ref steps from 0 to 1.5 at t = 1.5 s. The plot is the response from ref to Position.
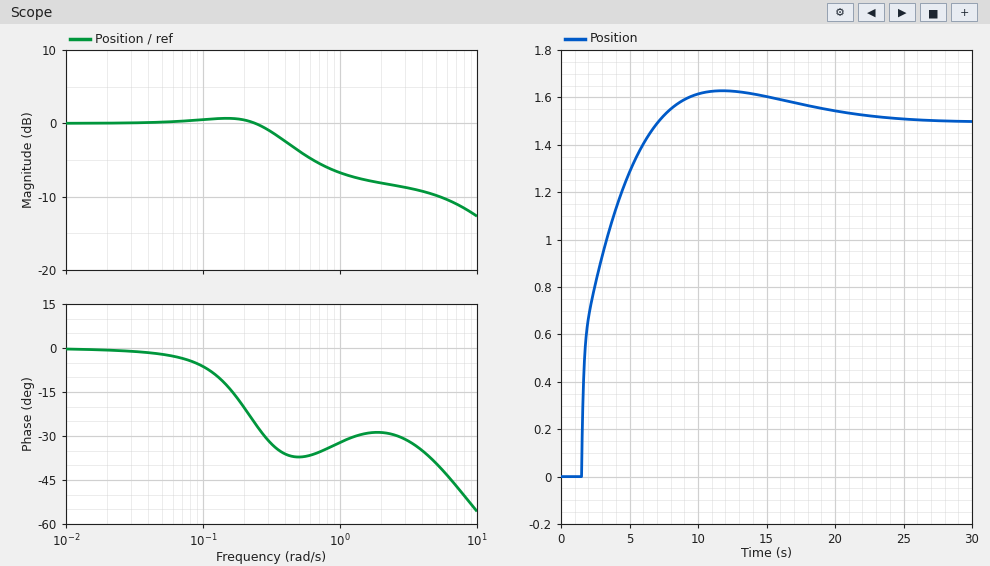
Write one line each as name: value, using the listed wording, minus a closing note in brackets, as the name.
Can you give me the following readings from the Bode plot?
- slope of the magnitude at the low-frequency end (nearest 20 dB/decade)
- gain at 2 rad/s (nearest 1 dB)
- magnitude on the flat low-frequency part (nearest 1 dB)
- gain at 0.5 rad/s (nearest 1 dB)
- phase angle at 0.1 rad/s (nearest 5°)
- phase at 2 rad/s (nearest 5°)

slope of the magnitude at the low-frequency end: 0 dB/decade
gain at 2 rad/s: -8 dB
magnitude on the flat low-frequency part: 0 dB
gain at 0.5 rad/s: -4 dB
phase angle at 0.1 rad/s: -5°
phase at 2 rad/s: -30°
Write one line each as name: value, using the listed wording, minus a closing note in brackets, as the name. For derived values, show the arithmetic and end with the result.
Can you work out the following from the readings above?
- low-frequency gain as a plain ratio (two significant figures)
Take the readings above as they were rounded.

low-frequency gain as a plain ratio: 10^(0 / 20) = 1.0
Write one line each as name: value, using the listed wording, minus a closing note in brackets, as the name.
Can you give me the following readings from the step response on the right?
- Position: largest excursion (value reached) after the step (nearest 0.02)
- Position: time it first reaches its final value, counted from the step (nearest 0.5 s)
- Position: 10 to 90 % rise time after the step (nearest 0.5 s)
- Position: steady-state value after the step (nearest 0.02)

Position: largest excursion (value reached) after the step: 1.62
Position: time it first reaches its final value, counted from the step: 5.5 s
Position: 10 to 90 % rise time after the step: 4.0 s
Position: steady-state value after the step: 1.50
